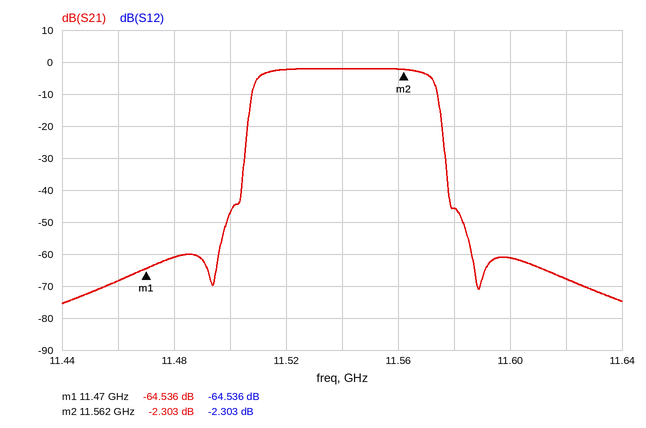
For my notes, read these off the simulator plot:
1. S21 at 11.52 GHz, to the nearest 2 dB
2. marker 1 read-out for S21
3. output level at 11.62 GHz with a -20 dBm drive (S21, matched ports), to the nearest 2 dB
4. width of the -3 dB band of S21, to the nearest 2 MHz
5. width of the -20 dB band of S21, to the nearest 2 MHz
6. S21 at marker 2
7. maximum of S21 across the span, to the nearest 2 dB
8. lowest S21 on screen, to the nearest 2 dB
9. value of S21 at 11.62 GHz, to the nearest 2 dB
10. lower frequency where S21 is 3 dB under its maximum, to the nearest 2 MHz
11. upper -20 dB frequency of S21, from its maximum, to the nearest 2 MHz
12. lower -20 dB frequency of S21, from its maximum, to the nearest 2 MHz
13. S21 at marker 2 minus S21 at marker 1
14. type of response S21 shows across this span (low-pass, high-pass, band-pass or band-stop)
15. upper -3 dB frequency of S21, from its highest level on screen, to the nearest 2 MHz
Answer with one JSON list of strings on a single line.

["-2 dB", "-64.536 dB", "-88 dBm", "62 MHz", "70 MHz", "-2.303 dB", "-2 dB", "-76 dB", "-68 dB", "11.510 GHz", "11.576 GHz", "11.506 GHz", "62.233 dB", "band-pass", "11.572 GHz"]
